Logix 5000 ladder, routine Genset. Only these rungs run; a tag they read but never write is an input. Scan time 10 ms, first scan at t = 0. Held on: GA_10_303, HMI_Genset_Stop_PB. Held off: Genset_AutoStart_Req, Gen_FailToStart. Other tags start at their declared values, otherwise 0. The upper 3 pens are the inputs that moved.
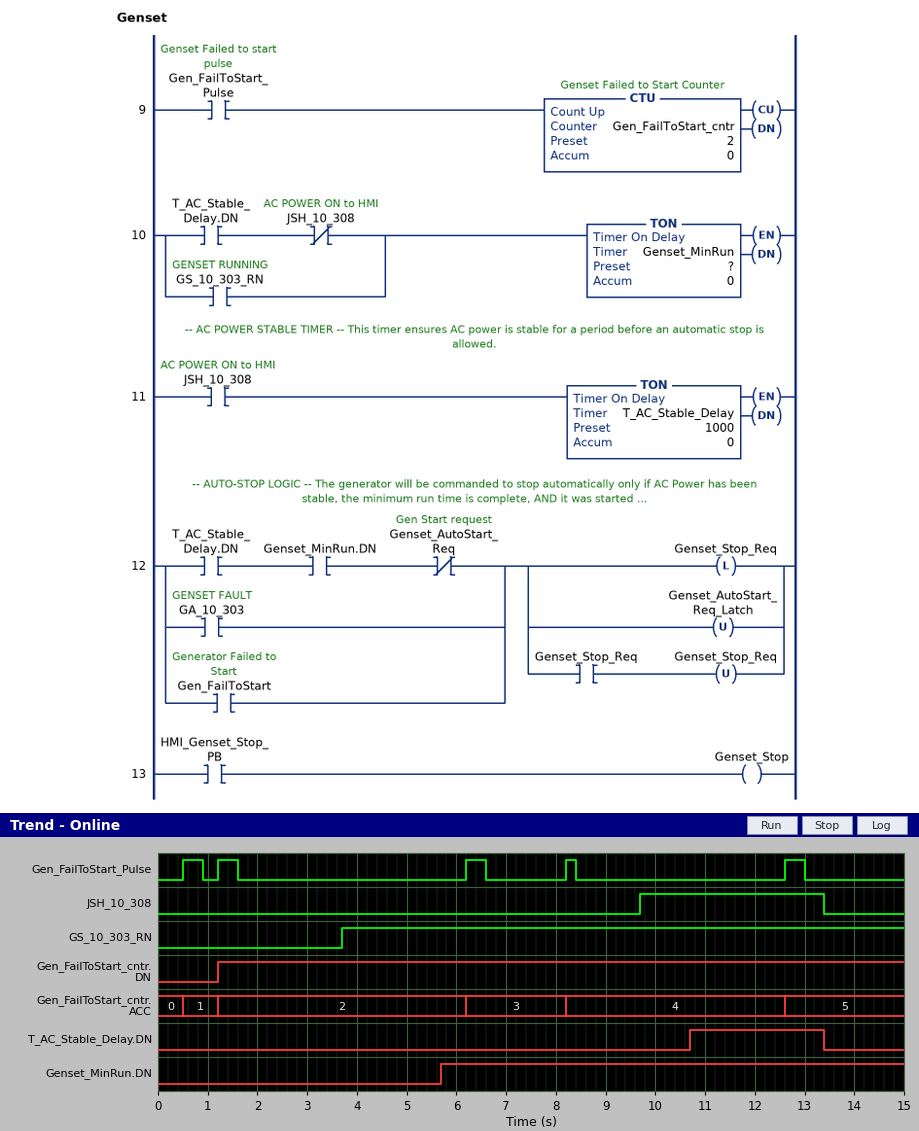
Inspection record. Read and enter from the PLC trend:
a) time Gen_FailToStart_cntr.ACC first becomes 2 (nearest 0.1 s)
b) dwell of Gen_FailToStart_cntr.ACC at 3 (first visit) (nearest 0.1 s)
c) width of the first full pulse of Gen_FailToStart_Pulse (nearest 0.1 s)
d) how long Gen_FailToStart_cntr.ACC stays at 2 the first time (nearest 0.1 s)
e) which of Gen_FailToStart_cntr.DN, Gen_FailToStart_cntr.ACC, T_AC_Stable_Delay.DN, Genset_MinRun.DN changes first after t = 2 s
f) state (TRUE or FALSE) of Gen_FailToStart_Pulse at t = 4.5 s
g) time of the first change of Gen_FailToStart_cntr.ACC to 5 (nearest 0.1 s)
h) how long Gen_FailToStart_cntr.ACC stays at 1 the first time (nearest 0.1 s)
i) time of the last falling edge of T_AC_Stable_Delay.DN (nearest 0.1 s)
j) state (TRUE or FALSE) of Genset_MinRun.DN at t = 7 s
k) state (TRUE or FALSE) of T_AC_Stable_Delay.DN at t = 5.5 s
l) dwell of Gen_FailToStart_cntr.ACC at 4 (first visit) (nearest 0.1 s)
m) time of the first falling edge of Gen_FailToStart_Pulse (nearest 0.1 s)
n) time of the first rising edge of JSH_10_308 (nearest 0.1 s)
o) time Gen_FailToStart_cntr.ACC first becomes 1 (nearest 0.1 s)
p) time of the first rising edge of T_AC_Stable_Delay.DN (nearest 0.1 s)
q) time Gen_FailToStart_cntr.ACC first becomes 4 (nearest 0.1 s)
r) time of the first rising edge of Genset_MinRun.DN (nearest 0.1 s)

1.2 s
2.0 s
0.4 s
5.0 s
Genset_MinRun.DN
FALSE
12.6 s
0.7 s
13.4 s
TRUE
FALSE
4.4 s
0.9 s
9.7 s
0.5 s
10.7 s
8.2 s
5.7 s
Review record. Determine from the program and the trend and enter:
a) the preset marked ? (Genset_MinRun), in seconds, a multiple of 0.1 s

2.0 s
